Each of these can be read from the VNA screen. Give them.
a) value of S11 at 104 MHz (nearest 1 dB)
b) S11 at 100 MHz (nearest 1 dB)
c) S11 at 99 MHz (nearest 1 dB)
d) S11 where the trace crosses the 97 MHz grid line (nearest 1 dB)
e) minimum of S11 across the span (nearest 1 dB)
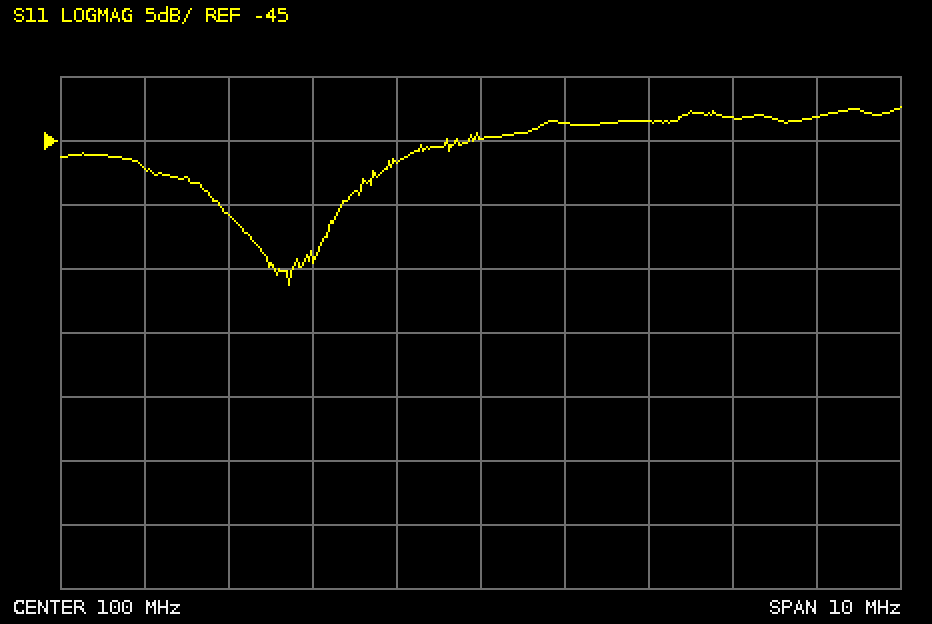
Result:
-43 dB
-45 dB
-47 dB
-51 dB
-56 dB
